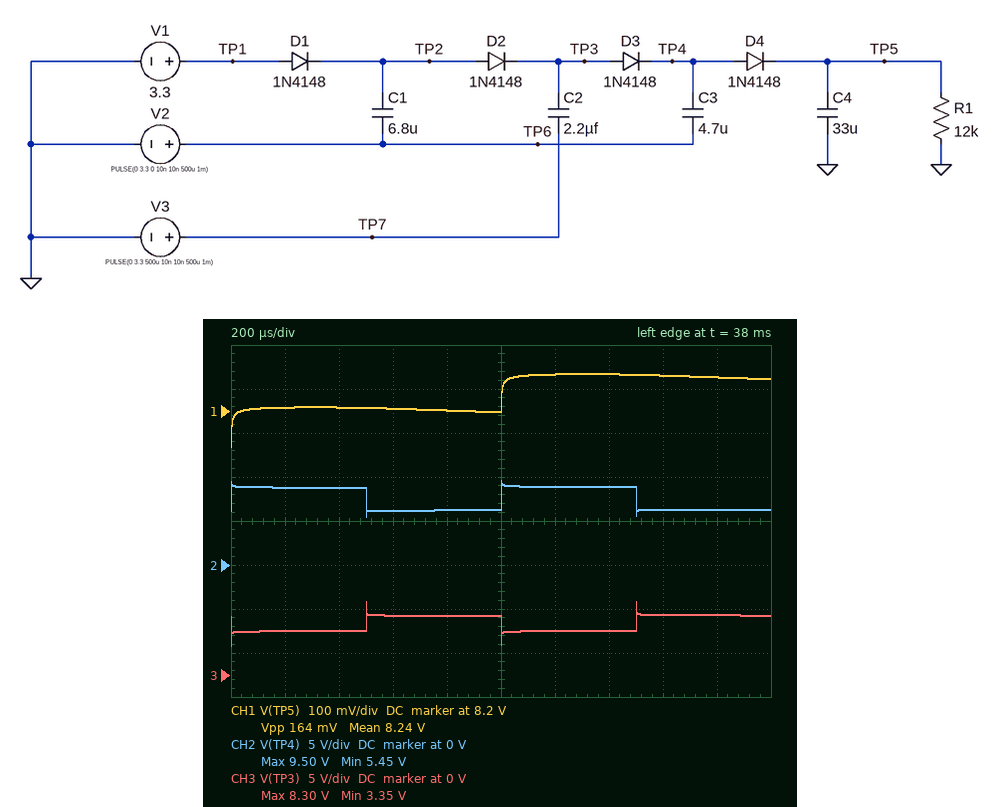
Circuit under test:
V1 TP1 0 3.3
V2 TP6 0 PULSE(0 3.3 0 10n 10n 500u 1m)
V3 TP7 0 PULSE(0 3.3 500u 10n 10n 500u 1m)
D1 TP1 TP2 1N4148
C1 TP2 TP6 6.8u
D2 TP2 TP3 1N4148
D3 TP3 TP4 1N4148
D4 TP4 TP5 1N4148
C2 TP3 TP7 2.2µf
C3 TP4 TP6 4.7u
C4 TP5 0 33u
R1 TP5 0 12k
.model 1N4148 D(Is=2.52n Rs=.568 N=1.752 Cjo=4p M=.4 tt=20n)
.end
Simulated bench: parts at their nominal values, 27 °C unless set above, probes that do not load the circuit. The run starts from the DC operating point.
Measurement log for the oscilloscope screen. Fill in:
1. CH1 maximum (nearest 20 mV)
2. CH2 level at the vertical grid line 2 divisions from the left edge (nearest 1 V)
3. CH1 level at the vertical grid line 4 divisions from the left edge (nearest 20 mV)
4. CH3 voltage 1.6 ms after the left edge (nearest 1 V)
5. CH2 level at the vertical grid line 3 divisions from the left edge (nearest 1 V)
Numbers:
8.28 V
9 V
8.20 V
7 V
6 V
